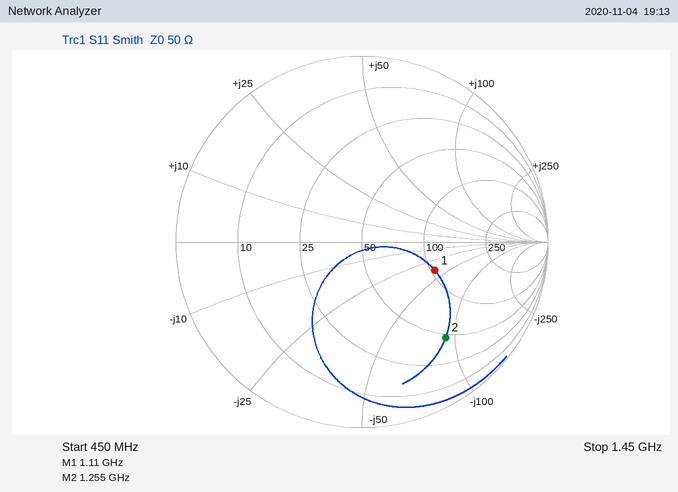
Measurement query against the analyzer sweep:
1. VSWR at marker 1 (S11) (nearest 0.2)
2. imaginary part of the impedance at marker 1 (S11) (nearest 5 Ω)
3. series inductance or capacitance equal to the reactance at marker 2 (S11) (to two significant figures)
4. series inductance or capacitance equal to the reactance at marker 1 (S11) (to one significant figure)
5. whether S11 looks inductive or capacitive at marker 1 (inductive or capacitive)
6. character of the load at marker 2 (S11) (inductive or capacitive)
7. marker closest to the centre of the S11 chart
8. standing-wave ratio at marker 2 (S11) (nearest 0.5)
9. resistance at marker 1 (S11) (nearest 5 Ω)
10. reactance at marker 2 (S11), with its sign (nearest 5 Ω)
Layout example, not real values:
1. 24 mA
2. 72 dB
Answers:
1. 2.4
2. -40 Ω
3. 1.4 pF
4. 4 pF
5. capacitive
6. capacitive
7. marker 1
8. 5.5
9. 105 Ω
10. -90 Ω
